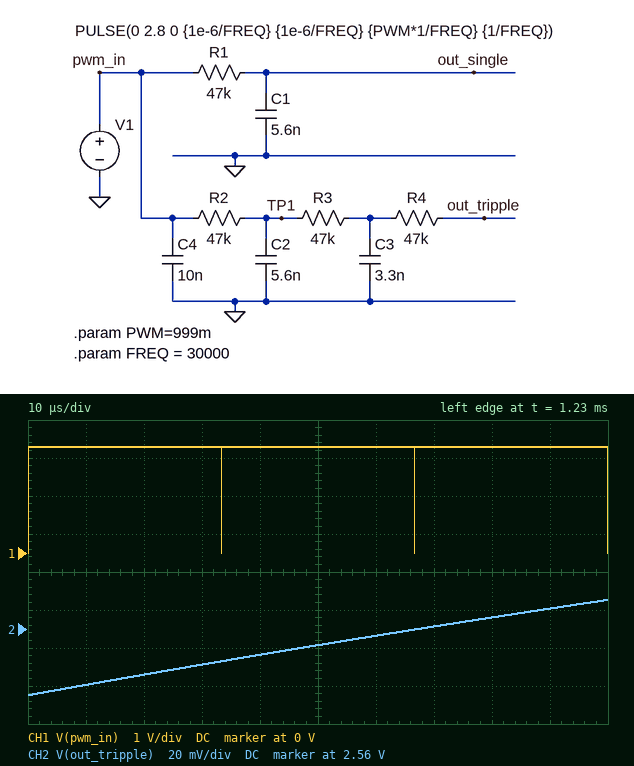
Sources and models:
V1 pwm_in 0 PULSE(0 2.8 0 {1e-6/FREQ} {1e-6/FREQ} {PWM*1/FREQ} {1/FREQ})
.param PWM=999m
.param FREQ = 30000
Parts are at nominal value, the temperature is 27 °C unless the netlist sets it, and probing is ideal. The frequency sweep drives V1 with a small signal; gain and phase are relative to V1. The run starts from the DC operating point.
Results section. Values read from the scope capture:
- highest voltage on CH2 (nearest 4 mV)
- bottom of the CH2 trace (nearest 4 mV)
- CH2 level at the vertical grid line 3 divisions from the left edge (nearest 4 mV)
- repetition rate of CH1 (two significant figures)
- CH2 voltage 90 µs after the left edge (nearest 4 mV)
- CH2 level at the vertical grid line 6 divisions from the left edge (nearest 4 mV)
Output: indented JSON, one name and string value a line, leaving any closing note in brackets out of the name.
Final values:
{
  "highest voltage on CH2": "2.576 V",
  "bottom of the CH2 trace": "2.524 V",
  "CH2 level at the vertical grid line 3 divisions from the left edge": "2.540 V",
  "repetition rate of CH1": "30 kHz",
  "CH2 voltage 90 µs after the left edge": "2.572 V",
  "CH2 level at the vertical grid line 6 divisions from the left edge": "2.556 V"
}
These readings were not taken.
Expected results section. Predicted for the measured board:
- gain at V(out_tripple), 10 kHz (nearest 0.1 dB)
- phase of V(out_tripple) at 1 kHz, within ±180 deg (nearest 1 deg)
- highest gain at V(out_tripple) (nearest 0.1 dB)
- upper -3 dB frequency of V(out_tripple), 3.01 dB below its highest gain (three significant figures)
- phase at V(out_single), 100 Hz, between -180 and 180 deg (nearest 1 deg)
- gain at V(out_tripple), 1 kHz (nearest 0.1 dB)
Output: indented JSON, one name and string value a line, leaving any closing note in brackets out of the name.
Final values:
{
  "gain at V(out_tripple), 10 kHz": "-44.3 dB",
  "phase of V(out_tripple) at 1 kHz, within ±180 deg": "-100 deg",
  "highest gain at V(out_tripple)": "0 dB",
  "upper -3 dB frequency of V(out_tripple), 3.01 dB below its highest gain": "316 Hz",
  "phase at V(out_single), 100 Hz, between -180 and 180 deg": "-9 deg",
  "gain at V(out_tripple), 1 kHz": "-11.3 dB"
}
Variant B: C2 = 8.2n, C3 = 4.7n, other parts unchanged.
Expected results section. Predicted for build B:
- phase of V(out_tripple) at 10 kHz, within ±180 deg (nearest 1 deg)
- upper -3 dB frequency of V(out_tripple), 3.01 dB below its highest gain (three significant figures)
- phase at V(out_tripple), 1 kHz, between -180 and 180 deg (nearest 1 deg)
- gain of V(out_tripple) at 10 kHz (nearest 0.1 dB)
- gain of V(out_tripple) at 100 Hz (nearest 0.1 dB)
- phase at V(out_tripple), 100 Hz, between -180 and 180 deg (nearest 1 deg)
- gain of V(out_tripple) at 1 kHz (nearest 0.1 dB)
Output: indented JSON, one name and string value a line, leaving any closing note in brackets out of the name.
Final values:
{
  "phase of V(out_tripple) at 10 kHz, within ±180 deg": "-171 deg",
  "upper -3 dB frequency of V(out_tripple), 3.01 dB below its highest gain": "219 Hz",
  "phase at V(out_tripple), 1 kHz, between -180 and 180 deg": "-114 deg",
  "gain of V(out_tripple) at 10 kHz": "-50.6 dB",
  "gain of V(out_tripple) at 100 Hz": "-0.8 dB",
  "phase at V(out_tripple), 100 Hz, between -180 and 180 deg": "-28 deg",
  "gain of V(out_tripple) at 1 kHz": "-15.1 dB"
}
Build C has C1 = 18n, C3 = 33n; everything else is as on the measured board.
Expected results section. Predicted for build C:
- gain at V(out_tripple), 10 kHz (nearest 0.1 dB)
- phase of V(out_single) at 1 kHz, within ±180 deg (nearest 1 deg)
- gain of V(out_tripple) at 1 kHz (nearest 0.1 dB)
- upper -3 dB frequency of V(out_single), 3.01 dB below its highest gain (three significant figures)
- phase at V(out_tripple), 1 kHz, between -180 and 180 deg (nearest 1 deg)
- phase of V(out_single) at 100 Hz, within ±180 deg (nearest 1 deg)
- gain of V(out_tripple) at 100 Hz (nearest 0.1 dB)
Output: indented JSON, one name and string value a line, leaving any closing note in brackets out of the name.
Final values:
{
  "gain at V(out_tripple), 10 kHz": "-64.2 dB",
  "phase of V(out_single) at 1 kHz, within ±180 deg": "-79 deg",
  "gain of V(out_tripple) at 1 kHz": "-28.3 dB",
  "upper -3 dB frequency of V(out_single), 3.01 dB below its highest gain": "188 Hz",
  "phase at V(out_tripple), 1 kHz, between -180 and 180 deg": "-126 deg",
  "phase of V(out_single) at 100 Hz, within ±180 deg": "-28 deg",
  "gain of V(out_tripple) at 100 Hz": "-7.1 dB"
}
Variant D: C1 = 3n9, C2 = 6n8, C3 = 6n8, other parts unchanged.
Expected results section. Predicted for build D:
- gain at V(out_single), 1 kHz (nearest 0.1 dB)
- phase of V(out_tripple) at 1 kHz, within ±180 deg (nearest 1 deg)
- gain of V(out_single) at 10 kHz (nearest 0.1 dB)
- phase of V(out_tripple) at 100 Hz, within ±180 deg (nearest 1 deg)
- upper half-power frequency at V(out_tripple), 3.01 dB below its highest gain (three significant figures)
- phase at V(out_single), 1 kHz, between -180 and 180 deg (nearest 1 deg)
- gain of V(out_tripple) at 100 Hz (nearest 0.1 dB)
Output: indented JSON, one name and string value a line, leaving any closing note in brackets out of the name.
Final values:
{
  "gain at V(out_single), 1 kHz": "-3.7 dB",
  "phase of V(out_tripple) at 1 kHz, within ±180 deg": "-117 deg",
  "gain of V(out_single) at 10 kHz": "-21.3 dB",
  "phase of V(out_tripple) at 100 Hz, within ±180 deg": "-32 deg",
  "upper half-power frequency at V(out_tripple), 3.01 dB below its highest gain": "186 Hz",
  "phase at V(out_single), 1 kHz, between -180 and 180 deg": "-49 deg",
  "gain of V(out_tripple) at 100 Hz": "-1.1 dB"
}
